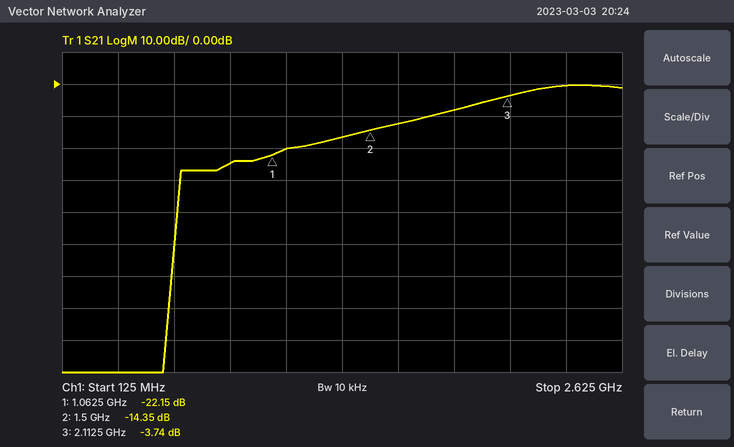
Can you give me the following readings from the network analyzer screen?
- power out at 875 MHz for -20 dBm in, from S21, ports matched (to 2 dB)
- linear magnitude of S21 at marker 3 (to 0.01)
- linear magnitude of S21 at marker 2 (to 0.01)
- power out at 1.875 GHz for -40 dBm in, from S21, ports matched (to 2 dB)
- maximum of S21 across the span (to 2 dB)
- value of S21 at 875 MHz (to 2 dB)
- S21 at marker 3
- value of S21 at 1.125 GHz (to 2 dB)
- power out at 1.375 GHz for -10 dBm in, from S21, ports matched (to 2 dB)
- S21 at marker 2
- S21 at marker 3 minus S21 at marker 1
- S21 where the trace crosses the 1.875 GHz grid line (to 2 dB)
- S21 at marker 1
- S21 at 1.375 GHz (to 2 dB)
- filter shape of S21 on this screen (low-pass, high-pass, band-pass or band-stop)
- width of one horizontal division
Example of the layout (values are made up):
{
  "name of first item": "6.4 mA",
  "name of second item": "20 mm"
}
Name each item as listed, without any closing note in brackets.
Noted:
{
  "power out at 875 MHz for -20 dBm in, from S21, ports matched": "-44 dBm",
  "linear magnitude of S21 at marker 3": "0.65",
  "linear magnitude of S21 at marker 2": "0.19",
  "power out at 1.875 GHz for -40 dBm in, from S21, ports matched": "-48 dBm",
  "maximum of S21 across the span": "0 dB",
  "value of S21 at 875 MHz": "-24 dB",
  "S21 at marker 3": "-3.74 dB",
  "value of S21 at 1.125 GHz": "-20 dB",
  "power out at 1.375 GHz for -10 dBm in, from S21, ports matched": "-26 dBm",
  "S21 at marker 2": "-14.35 dB",
  "S21 at marker 3 minus S21 at marker 1": "18.41 dB",
  "S21 where the trace crosses the 1.875 GHz grid line": "-8 dB",
  "S21 at marker 1": "-22.15 dB",
  "S21 at 1.375 GHz": "-16 dB",
  "filter shape of S21 on this screen": "high-pass",
  "width of one horizontal division": "250 MHz"
}
